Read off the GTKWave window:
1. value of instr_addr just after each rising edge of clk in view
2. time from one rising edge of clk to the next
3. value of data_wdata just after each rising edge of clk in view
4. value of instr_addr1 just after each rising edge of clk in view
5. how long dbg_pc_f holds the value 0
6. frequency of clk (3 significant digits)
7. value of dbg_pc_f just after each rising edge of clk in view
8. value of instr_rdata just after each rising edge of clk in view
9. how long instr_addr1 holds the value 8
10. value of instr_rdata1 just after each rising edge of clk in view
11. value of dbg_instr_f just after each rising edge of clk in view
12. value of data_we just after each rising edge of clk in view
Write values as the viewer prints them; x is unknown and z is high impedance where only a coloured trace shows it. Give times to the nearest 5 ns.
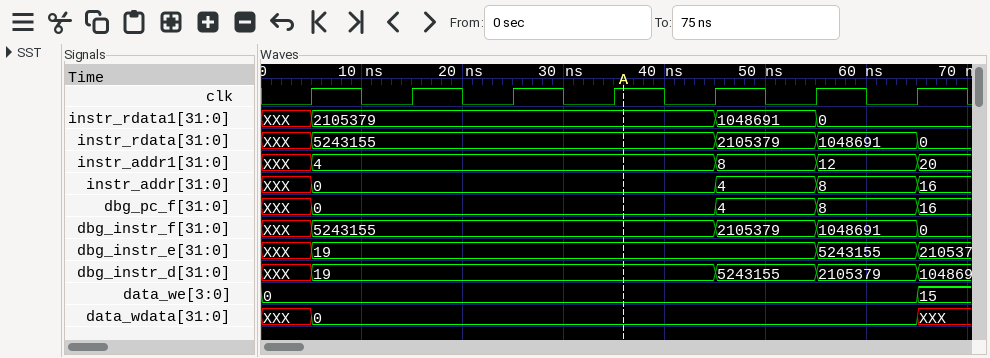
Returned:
0, 0, 0, 0, 4, 8, 16
10 ns
0, 0, 0, 0, 0, 0, XXX
4, 4, 4, 4, 8, 12, 20
40 ns
100 MHz
0, 0, 0, 0, 4, 8, 16
5243155, 5243155, 5243155, 5243155, 2105379, 1048691, 0
10 ns
2105379, 2105379, 2105379, 2105379, 1048691, 0, 0
5243155, 5243155, 5243155, 5243155, 2105379, 1048691, 0
0, 0, 0, 0, 0, 0, 15
